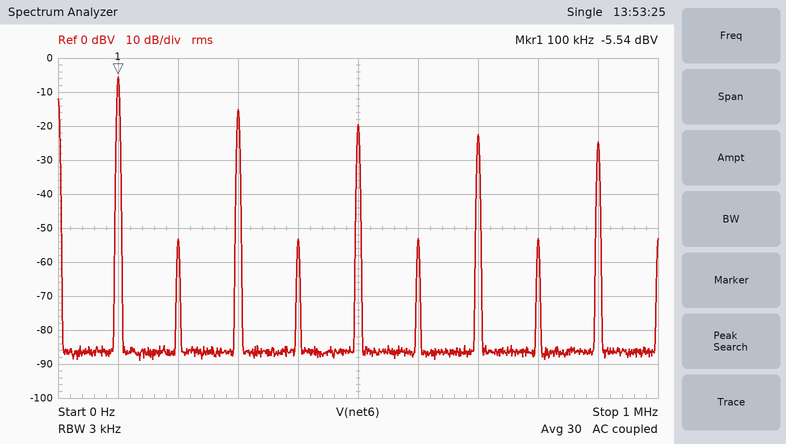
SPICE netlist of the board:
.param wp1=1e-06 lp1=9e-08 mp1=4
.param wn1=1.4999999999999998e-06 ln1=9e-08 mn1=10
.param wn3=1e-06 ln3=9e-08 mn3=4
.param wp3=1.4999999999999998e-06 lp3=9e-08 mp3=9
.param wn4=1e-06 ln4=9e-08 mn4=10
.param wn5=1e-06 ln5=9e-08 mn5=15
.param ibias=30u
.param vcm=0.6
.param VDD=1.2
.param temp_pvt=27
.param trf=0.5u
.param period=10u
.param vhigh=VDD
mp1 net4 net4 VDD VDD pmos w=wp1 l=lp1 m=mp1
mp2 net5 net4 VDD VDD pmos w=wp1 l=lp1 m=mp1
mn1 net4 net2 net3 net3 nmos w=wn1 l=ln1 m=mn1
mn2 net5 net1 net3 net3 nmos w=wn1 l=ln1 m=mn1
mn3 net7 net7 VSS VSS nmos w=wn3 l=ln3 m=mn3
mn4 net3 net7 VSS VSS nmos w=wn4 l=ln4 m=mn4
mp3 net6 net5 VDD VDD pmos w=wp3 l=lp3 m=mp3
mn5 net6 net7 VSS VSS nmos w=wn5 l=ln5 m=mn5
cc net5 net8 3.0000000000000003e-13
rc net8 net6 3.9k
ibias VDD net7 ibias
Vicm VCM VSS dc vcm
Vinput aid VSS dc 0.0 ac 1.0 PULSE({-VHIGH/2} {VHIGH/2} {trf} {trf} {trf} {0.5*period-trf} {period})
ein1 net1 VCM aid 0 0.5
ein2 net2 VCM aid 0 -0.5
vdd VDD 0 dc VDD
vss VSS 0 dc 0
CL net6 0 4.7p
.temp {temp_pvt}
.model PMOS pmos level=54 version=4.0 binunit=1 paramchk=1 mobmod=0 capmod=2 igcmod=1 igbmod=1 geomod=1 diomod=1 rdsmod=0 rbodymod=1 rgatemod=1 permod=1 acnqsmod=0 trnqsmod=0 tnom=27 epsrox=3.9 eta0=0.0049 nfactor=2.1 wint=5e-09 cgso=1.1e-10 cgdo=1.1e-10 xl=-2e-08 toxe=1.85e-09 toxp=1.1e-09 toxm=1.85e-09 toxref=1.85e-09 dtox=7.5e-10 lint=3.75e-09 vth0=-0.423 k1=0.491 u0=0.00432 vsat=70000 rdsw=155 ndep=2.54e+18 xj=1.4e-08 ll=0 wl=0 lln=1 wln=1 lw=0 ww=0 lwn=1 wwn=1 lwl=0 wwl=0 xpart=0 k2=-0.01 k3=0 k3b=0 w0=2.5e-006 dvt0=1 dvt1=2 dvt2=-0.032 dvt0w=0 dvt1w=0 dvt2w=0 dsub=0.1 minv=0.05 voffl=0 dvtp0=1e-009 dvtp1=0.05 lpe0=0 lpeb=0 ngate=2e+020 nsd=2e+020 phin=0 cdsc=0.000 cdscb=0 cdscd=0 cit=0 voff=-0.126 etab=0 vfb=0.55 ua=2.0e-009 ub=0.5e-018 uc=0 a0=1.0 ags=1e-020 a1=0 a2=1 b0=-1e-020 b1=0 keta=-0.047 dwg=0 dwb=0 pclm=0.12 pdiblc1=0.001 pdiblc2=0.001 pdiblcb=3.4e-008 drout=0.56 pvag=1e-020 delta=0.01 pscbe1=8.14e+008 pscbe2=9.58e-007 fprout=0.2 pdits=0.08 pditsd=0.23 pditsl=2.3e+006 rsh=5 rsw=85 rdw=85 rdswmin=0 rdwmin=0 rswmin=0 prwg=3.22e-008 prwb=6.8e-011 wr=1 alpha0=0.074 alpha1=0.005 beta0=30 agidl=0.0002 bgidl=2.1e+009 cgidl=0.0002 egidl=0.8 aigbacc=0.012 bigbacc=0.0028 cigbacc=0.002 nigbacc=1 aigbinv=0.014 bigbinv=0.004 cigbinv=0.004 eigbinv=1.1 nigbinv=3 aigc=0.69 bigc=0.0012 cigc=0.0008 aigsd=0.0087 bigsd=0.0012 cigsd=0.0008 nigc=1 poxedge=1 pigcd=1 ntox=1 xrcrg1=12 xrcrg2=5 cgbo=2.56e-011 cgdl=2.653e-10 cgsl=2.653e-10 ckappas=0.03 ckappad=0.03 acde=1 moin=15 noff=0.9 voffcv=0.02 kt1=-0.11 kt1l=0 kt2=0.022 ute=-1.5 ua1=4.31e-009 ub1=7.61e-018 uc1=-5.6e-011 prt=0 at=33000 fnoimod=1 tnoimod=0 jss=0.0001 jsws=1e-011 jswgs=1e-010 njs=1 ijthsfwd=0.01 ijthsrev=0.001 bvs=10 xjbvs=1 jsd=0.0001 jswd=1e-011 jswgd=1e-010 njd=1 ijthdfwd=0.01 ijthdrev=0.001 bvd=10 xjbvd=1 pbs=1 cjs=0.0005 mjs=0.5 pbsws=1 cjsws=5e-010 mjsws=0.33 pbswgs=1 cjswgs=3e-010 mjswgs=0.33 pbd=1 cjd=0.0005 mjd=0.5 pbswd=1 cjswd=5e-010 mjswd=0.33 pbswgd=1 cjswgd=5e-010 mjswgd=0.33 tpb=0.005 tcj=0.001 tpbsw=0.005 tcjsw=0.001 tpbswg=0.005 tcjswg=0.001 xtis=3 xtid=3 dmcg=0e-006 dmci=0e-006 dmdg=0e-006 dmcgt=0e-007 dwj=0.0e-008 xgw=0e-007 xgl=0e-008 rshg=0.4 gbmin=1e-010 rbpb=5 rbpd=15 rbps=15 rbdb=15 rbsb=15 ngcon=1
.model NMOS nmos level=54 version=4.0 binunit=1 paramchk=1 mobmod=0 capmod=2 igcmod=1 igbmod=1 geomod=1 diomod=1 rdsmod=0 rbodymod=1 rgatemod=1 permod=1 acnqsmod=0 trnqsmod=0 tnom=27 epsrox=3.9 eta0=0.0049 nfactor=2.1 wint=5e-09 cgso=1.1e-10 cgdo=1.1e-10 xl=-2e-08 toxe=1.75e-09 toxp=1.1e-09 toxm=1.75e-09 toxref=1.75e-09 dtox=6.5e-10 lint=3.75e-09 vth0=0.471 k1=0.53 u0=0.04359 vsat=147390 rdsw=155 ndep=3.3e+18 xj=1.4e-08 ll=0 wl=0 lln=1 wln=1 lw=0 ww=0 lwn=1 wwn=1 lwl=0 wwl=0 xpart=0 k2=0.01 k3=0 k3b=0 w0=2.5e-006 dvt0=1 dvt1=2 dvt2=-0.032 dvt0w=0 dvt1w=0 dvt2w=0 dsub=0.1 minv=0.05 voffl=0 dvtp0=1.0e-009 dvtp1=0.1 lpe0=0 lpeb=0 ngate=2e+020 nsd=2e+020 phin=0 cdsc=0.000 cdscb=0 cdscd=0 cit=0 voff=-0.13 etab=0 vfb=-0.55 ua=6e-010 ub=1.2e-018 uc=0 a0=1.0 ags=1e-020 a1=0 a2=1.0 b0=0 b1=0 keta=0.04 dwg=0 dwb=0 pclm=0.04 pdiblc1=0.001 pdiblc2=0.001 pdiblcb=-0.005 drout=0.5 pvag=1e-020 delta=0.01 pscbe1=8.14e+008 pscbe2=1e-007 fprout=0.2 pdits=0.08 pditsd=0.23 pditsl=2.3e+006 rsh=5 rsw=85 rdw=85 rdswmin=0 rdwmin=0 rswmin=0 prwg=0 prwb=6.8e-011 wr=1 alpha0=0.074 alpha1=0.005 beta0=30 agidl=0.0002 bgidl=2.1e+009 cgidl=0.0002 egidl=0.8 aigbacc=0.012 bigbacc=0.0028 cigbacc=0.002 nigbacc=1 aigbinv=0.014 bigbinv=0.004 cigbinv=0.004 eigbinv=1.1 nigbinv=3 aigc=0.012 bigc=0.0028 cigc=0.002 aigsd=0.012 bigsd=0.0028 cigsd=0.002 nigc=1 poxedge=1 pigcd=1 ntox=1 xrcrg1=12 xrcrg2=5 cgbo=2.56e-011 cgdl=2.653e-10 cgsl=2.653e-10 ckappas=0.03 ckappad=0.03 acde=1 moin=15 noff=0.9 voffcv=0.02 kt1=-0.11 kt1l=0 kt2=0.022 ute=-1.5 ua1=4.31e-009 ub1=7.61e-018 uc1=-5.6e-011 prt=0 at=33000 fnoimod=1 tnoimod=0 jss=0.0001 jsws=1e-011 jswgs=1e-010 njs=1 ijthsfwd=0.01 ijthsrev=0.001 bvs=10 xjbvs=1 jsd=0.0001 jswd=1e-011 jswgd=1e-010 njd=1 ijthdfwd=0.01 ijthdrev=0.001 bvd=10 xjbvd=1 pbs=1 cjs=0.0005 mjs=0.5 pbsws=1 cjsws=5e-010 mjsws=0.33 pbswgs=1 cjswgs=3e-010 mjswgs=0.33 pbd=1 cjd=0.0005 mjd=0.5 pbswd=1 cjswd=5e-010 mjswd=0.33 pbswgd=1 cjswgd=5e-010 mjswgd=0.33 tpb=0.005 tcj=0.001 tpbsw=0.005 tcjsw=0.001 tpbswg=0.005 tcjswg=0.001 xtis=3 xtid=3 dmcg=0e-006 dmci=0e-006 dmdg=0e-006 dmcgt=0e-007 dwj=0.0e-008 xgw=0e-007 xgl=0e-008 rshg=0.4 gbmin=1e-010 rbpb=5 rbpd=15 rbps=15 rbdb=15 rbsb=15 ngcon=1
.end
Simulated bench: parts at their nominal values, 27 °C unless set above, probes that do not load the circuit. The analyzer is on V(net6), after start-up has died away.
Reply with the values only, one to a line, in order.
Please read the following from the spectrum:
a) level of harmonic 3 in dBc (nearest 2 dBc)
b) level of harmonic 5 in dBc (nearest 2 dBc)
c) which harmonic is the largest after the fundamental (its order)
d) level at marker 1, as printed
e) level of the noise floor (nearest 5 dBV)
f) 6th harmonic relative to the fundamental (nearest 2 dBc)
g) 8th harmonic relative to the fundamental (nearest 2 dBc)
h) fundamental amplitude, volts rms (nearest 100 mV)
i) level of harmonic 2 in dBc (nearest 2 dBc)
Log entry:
-10 dBc
-14 dBc
3
-5.54 dBV
-85 dBV
-48 dBc
-48 dBc
500 mV
-48 dBc
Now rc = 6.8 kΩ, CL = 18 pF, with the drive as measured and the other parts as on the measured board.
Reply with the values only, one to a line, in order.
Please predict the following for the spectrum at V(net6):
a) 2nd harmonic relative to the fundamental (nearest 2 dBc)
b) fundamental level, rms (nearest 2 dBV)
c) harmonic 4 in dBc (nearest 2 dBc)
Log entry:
-34 dBc
-6 dBV
-34 dBc
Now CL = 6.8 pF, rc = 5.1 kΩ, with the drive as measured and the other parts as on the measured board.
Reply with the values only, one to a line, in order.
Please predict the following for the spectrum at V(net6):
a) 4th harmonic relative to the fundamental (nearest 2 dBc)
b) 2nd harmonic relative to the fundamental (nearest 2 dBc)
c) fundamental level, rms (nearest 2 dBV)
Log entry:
-44 dBc
-44 dBc
-6 dBV
